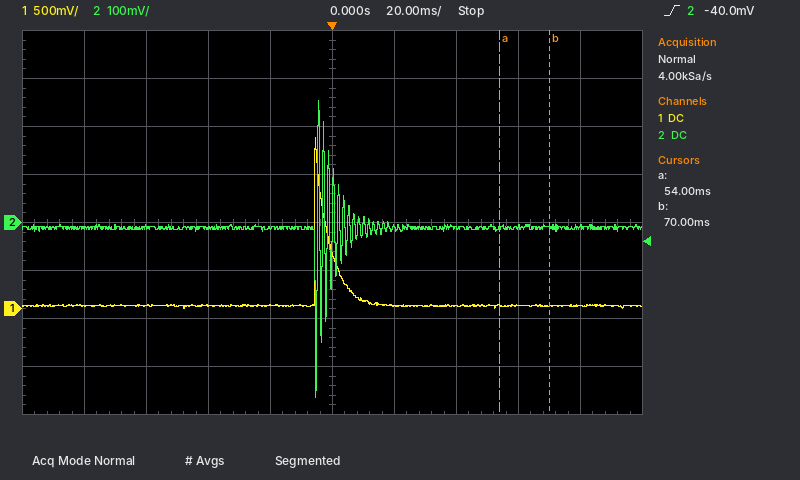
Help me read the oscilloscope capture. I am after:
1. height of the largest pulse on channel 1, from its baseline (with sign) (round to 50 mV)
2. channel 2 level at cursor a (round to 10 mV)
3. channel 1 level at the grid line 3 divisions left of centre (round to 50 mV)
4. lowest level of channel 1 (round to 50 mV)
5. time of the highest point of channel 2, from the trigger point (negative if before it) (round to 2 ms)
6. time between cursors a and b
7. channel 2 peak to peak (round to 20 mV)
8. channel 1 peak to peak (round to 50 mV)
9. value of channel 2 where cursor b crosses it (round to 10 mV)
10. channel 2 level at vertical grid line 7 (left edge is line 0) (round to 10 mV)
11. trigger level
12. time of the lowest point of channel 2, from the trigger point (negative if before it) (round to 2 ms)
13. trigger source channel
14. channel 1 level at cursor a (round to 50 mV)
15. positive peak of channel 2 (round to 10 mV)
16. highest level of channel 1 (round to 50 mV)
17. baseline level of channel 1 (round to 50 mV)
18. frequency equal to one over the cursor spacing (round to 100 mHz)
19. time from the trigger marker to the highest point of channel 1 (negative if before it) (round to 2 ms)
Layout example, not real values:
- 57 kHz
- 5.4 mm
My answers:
- +1.75 V
- -10 mV
- 50 mV
- 0 mV
- -4 ms
- 16 ms
- 620 mV
- 1.80 V
- -10 mV
- -10 mV
- -40.0 mV
- -6 ms
- channel 2
- 50 mV
- 250 mV
- 1.80 V
- 50 mV
- 62.5 Hz
- -6 ms
